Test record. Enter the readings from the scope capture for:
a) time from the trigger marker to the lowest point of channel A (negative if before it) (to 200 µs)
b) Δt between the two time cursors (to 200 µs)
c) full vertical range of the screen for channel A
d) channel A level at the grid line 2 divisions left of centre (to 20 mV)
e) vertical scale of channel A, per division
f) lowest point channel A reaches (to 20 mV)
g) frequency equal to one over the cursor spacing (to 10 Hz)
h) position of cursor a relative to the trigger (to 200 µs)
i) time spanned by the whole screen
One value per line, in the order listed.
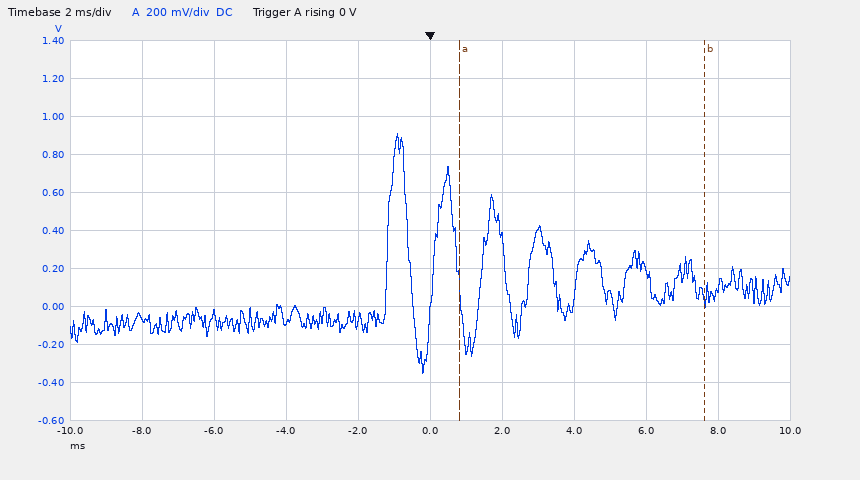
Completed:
-200 µs
6.8 ms
2 V
-80 mV
200 mV
-360 mV
150 Hz
+800 µs
20 ms
